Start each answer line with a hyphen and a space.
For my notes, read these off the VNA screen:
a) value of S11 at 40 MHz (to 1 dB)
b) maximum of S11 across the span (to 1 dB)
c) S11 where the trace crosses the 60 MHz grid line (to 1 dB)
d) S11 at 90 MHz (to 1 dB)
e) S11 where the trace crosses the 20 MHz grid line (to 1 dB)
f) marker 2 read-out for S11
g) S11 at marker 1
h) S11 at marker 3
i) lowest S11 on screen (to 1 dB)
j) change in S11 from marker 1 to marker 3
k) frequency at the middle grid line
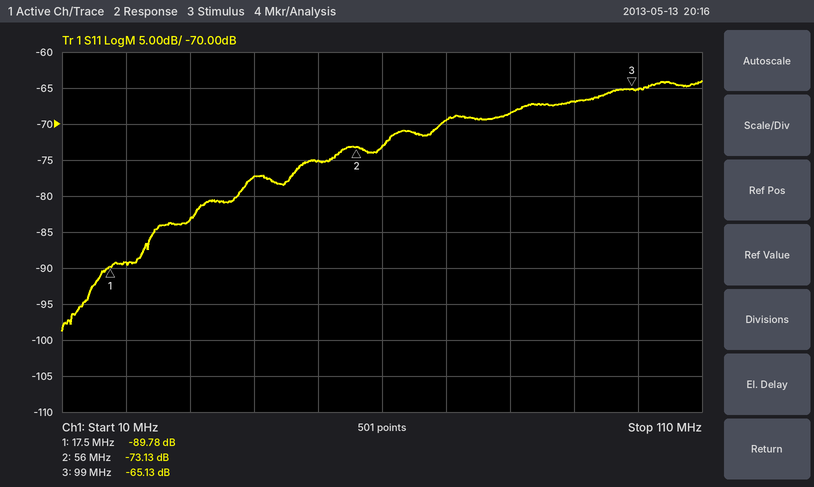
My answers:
- -77 dB
- -64 dB
- -73 dB
- -67 dB
- -89 dB
- -73.13 dB
- -89.78 dB
- -65.13 dB
- -99 dB
- 24.65 dB
- 60 MHz
